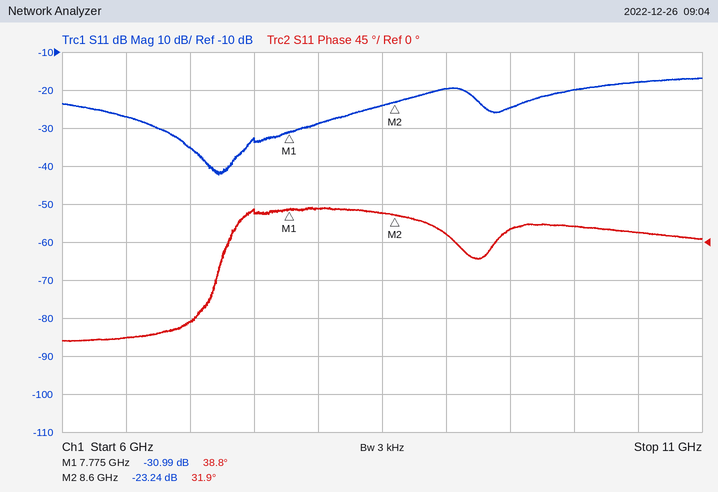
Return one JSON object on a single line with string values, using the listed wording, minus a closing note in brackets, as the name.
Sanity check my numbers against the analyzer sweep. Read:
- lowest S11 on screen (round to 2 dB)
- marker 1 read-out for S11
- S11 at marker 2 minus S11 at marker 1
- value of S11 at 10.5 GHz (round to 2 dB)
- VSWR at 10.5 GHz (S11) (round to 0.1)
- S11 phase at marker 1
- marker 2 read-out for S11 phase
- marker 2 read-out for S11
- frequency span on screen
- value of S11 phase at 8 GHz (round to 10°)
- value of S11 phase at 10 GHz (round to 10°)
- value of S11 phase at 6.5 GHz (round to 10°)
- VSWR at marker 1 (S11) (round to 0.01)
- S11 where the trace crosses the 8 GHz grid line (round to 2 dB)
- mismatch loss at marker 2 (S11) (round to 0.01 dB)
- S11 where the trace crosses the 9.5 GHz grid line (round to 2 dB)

{"lowest S11 on screen": "-42 dB", "marker 1 read-out for S11": "-30.99 dB", "S11 at marker 2 minus S11 at marker 1": "7.75 dB", "value of S11 at 10.5 GHz": "-18 dB", "VSWR at 10.5 GHz (S11)": "1.3", "S11 phase at marker 1": "38.8°", "marker 2 read-out for S11 phase": "31.9°", "marker 2 read-out for S11": "-23.24 dB", "frequency span on screen": "5 GHz", "value of S11 phase at 8 GHz": "40°", "value of S11 phase at 10 GHz": "20°", "value of S11 phase at 6.5 GHz": "-110°", "VSWR at marker 1 (S11)": "1.06", "S11 where the trace crosses the 8 GHz grid line": "-28 dB", "mismatch loss at marker 2 (S11)": "0.02 dB", "S11 where the trace crosses the 9.5 GHz grid line": "-24 dB"}
